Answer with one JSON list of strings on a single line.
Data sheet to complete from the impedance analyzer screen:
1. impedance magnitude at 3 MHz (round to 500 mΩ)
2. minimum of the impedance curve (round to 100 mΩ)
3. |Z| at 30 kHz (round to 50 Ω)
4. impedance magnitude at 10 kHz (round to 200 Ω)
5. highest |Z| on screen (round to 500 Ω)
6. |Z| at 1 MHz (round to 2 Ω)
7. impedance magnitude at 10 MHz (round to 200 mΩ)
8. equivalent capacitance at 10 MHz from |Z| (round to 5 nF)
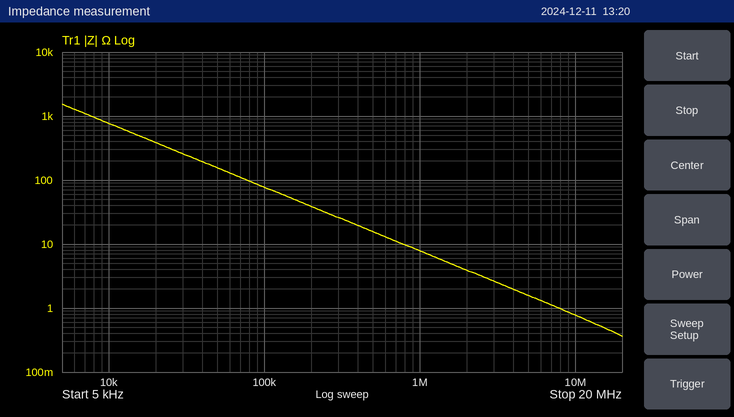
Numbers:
["2.5 Ω", "400 mΩ", "250 Ω", "800 Ω", "1.5 kΩ", "8 Ω", "800 mΩ", "20 nF"]
